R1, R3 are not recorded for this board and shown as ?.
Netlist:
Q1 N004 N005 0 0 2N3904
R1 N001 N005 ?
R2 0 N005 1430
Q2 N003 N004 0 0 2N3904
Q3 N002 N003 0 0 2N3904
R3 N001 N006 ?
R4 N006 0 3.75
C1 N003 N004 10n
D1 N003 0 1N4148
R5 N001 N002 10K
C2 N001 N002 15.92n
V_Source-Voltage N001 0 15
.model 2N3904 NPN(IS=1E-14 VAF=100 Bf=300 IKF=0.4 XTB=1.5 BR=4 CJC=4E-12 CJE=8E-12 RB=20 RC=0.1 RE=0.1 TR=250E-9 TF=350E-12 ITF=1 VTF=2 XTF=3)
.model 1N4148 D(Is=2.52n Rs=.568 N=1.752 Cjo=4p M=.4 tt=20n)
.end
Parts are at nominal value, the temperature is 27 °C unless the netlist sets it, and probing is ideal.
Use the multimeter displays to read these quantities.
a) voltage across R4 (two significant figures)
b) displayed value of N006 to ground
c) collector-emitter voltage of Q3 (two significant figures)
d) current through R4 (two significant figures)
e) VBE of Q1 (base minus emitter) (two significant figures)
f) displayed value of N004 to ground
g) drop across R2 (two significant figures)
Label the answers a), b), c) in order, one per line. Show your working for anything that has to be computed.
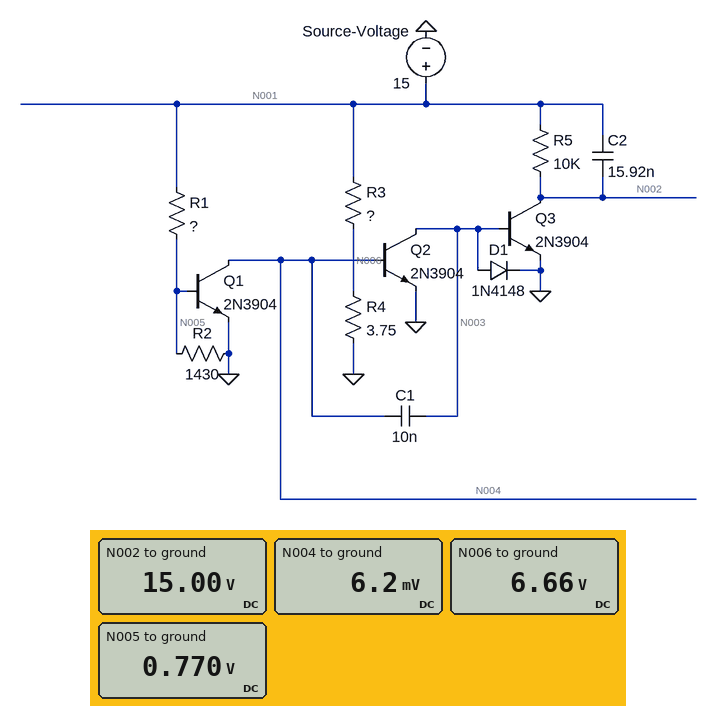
a) 6.66 V = 6.7 V
b) 6.66 V
c) 15 V = 15 V
d) (6.66 V) / 3.75 Ω = 1.8 A
e) 770 mV = 770 mV
f) 6.2 mV
g) 770 mV = 770 mV
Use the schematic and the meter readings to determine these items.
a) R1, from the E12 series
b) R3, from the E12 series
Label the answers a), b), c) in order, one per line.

a) 4.7 kΩ
b) 4.7 Ω
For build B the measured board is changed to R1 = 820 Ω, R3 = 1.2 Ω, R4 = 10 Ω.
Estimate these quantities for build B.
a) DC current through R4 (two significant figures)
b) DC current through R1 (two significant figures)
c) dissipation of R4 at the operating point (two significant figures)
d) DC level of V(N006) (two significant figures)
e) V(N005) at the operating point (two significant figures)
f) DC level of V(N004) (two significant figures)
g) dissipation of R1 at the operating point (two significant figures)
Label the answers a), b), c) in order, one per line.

a) 1.3 A
b) 17 mA
c) 18 W
d) 13 V
e) 1.1 V
f) 8.3 mV
g) 240 mW
